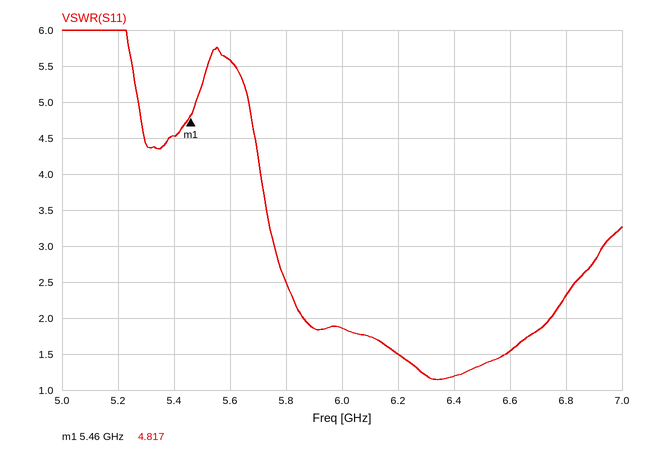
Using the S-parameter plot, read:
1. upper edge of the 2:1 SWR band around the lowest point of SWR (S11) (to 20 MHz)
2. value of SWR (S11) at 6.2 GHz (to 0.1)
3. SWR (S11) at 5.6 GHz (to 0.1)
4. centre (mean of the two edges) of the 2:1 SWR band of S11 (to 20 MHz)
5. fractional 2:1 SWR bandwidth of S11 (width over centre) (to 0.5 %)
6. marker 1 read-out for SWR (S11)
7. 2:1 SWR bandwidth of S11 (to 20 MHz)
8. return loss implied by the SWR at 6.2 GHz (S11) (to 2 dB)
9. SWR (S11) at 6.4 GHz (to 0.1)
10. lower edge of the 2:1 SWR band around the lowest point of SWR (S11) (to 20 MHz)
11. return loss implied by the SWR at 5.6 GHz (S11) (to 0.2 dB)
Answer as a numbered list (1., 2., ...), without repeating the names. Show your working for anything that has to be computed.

1. 6.74 GHz
2. 1.5
3. 5.6
4. 6.30 GHz
5. 880 MHz / 6.3 GHz ≈ 14.0 %
6. 4.817
7. 6.74 GHz − 5.86 GHz = 880 MHz
8. −20 log10((1.5 − 1)/(1.5 + 1)) ≈ 14 dB
9. 1.2
10. 5.86 GHz
11. −20 log10((5.6 − 1)/(5.6 + 1)) ≈ 3.14 dB, so 3.2 dB to the nearest 0.2 dB
